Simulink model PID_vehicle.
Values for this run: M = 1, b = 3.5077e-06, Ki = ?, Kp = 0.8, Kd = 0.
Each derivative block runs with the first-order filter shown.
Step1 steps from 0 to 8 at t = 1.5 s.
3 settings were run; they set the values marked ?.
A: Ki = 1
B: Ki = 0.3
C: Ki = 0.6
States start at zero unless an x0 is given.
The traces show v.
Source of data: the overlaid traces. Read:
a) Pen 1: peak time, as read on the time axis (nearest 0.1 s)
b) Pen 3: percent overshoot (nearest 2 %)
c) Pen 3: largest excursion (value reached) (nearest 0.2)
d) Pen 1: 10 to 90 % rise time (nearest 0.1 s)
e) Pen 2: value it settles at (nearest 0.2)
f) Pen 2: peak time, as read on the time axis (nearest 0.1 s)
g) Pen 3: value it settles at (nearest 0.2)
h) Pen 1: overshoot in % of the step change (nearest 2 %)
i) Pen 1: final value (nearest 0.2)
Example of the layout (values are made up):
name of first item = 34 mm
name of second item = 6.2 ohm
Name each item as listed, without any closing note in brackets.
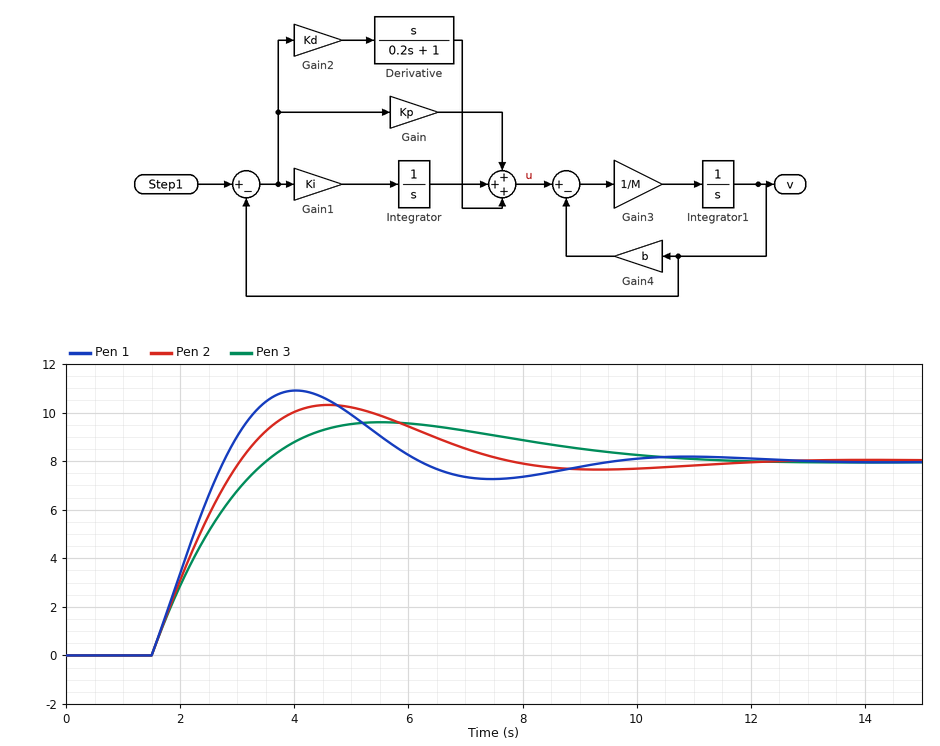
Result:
Pen 1: peak time, as read on the time axis = 4.0 s
Pen 3: percent overshoot = 20 %
Pen 3: largest excursion (value reached) = 9.6
Pen 1: 10 to 90 % rise time = 1.0 s
Pen 2: value it settles at = 8.0
Pen 2: peak time, as read on the time axis = 4.6 s
Pen 3: value it settles at = 8.0
Pen 1: overshoot in % of the step change = 36 %
Pen 1: final value = 8.0
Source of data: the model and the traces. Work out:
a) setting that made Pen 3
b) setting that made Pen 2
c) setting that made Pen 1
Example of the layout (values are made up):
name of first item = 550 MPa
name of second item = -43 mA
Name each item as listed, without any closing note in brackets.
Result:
setting that made Pen 3 = B
setting that made Pen 2 = C
setting that made Pen 1 = A
